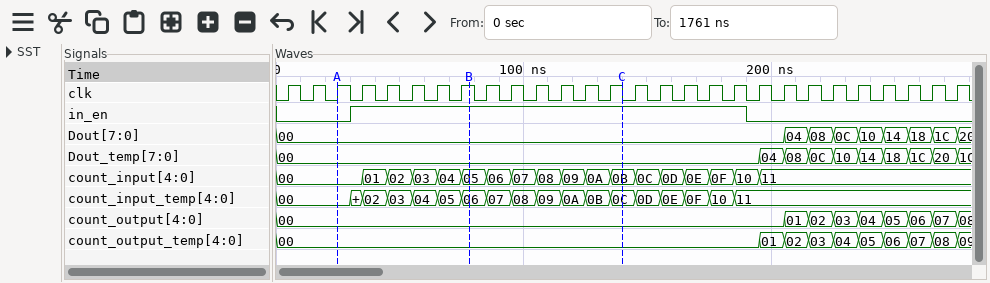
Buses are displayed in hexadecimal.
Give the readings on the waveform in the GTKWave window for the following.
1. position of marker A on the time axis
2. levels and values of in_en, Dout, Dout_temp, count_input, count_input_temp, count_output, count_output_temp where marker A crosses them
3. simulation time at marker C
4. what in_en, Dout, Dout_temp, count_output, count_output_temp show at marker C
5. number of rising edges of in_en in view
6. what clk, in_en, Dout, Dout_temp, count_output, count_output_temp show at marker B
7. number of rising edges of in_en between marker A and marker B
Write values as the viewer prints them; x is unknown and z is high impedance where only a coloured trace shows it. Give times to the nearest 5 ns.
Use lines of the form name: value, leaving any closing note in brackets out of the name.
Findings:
position of marker A on the time axis: 25 ns
levels and values of in_en, Dout, Dout_temp, count_input, count_input_temp, count_output, count_output_temp where marker A crosses them: in_en=0, Dout=00, Dout_temp=00, count_input=00, count_input_temp=00, count_output=00, count_output_temp=00
simulation time at marker C: 140 ns
what in_en, Dout, Dout_temp, count_output, count_output_temp show at marker C: in_en=1, Dout=00, Dout_temp=00, count_output=00, count_output_temp=00
number of rising edges of in_en in view: 1
what clk, in_en, Dout, Dout_temp, count_output, count_output_temp show at marker B: clk=1, in_en=1, Dout=00, Dout_temp=00, count_output=00, count_output_temp=00
number of rising edges of in_en between marker A and marker B: 1
